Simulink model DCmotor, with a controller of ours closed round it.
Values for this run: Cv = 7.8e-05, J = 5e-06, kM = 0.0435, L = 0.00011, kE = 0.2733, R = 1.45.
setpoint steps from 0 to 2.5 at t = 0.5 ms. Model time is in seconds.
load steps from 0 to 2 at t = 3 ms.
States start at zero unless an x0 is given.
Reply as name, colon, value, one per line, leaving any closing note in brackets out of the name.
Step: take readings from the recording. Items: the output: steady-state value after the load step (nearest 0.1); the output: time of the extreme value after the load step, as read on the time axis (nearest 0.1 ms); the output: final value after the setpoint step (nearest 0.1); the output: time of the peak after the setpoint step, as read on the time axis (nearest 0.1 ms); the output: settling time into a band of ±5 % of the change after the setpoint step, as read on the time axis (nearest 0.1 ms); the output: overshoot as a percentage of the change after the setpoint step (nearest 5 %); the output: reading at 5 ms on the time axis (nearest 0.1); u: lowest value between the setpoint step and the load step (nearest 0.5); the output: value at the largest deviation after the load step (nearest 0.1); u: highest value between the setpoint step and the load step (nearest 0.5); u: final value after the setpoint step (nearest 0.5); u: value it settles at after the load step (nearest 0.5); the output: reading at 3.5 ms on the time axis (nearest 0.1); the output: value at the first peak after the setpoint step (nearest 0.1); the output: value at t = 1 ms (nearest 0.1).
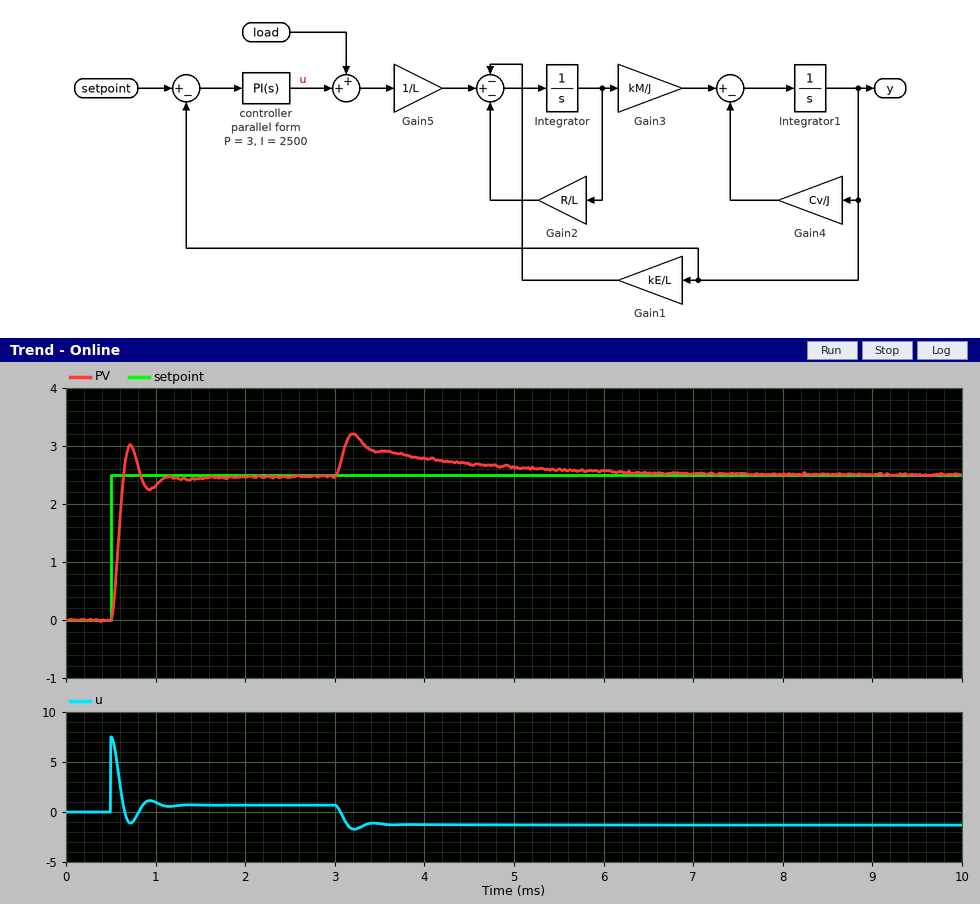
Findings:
the output: steady-state value after the load step: 2.5
the output: time of the extreme value after the load step, as read on the time axis: 3.2 ms
the output: final value after the setpoint step: 2.5
the output: time of the peak after the setpoint step, as read on the time axis: 0.7 ms
the output: settling time into a band of ±5 % of the change after the setpoint step, as read on the time axis: 1.0 ms
the output: overshoot as a percentage of the change after the setpoint step: 20 %
the output: reading at 5 ms on the time axis: 2.6
u: lowest value between the setpoint step and the load step: -1.0
the output: value at the largest deviation after the load step: 3.2
u: highest value between the setpoint step and the load step: 7.5
u: final value after the setpoint step: 0.5
u: value it settles at after the load step: -1.5
the output: reading at 3.5 ms on the time axis: 2.9
the output: value at the first peak after the setpoint step: 3.0
the output: value at t = 1 ms: 2.3
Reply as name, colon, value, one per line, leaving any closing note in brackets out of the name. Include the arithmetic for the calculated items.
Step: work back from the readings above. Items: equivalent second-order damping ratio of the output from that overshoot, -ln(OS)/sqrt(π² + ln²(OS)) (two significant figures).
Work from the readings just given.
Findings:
equivalent second-order damping ratio of the output from that overshoot, -ln(OS)/sqrt(π² + ln²(OS)): ln(0.2) = -1.609; 1.609 / sqrt(9.870 + 2.590) = 0.46
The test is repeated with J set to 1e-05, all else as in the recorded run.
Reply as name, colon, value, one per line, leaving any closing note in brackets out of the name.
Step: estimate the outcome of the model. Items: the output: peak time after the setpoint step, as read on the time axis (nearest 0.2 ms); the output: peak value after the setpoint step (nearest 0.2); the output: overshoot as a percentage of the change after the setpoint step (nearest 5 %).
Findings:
the output: peak time after the setpoint step, as read on the time axis: 0.8 ms
the output: peak value after the setpoint step: 2.8
the output: overshoot as a percentage of the change after the setpoint step: 10 %
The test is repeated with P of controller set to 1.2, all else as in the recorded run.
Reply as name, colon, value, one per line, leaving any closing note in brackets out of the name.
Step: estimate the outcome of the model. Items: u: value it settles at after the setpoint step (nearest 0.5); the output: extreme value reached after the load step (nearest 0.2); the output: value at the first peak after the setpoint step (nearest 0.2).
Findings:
u: value it settles at after the setpoint step: 0.5
the output: extreme value reached after the load step: 3.8
the output: value at the first peak after the setpoint step: 2.8
